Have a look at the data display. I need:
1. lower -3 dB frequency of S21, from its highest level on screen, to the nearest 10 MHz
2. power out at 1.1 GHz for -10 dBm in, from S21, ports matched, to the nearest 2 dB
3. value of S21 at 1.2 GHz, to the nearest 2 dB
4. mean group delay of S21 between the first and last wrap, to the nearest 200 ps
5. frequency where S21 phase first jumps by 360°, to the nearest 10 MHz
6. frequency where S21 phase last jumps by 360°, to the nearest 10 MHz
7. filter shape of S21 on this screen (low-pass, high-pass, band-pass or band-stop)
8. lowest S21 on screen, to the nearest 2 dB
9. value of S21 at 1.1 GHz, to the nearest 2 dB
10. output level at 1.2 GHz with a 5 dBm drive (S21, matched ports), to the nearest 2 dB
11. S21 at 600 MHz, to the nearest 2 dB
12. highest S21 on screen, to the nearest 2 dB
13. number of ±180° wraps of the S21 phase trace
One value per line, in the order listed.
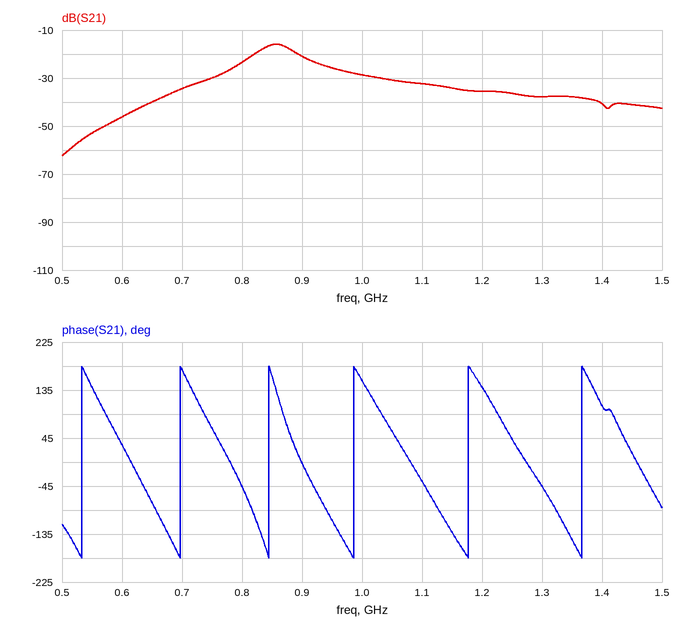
830 MHz
-42 dBm
-36 dB
6.0 ns
530 MHz
1.37 GHz
band-pass
-62 dB
-32 dB
-30 dBm
-46 dB
-16 dB
6
